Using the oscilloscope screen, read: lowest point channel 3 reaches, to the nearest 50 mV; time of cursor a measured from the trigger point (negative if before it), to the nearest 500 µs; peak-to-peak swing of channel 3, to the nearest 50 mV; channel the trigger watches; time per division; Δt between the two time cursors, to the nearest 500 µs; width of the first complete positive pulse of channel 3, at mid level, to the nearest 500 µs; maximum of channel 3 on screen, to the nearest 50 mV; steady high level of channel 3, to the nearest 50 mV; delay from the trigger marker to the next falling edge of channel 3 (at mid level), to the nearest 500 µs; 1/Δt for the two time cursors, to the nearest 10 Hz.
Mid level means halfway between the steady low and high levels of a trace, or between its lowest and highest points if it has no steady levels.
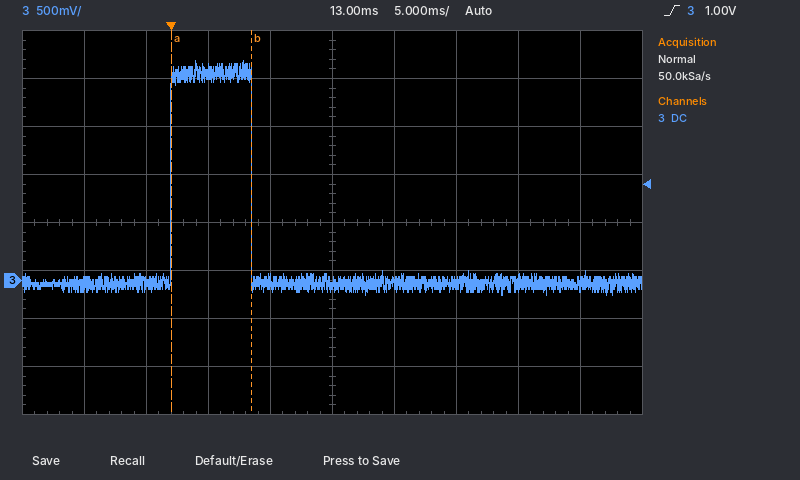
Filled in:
-150 mV
0.0 ms
2.45 V
channel 3
5 ms
6.5 ms
6.5 ms
2.30 V
2.15 V
6.5 ms
150 Hz
